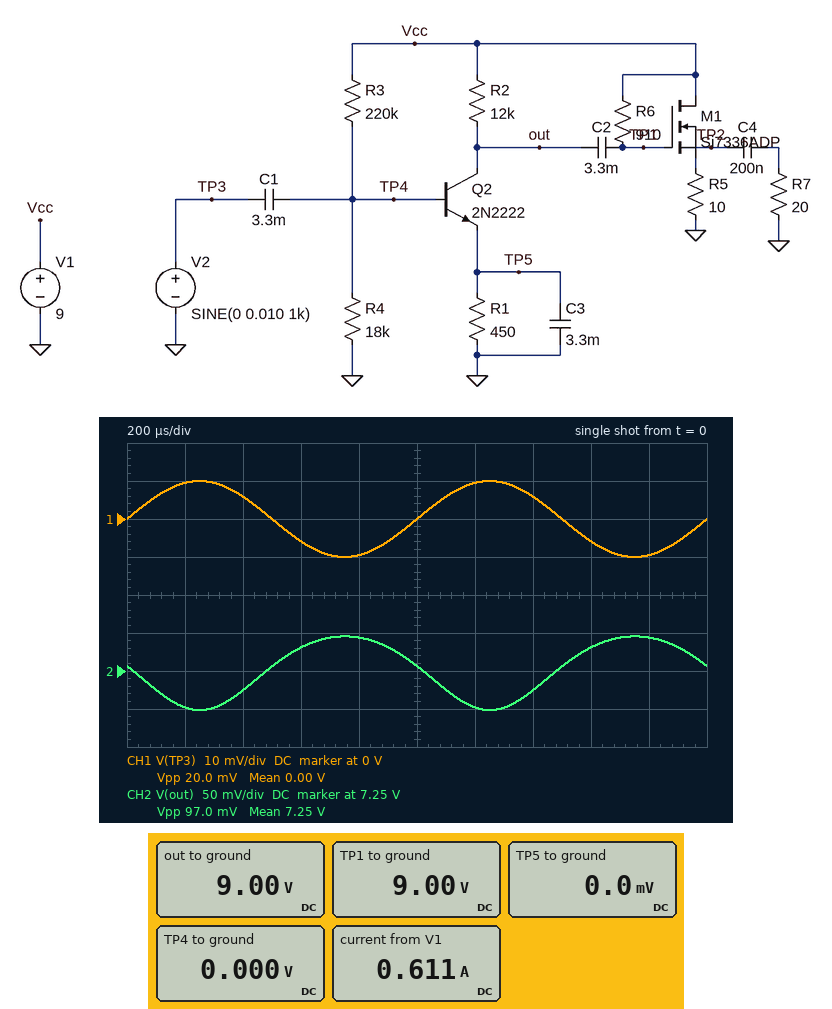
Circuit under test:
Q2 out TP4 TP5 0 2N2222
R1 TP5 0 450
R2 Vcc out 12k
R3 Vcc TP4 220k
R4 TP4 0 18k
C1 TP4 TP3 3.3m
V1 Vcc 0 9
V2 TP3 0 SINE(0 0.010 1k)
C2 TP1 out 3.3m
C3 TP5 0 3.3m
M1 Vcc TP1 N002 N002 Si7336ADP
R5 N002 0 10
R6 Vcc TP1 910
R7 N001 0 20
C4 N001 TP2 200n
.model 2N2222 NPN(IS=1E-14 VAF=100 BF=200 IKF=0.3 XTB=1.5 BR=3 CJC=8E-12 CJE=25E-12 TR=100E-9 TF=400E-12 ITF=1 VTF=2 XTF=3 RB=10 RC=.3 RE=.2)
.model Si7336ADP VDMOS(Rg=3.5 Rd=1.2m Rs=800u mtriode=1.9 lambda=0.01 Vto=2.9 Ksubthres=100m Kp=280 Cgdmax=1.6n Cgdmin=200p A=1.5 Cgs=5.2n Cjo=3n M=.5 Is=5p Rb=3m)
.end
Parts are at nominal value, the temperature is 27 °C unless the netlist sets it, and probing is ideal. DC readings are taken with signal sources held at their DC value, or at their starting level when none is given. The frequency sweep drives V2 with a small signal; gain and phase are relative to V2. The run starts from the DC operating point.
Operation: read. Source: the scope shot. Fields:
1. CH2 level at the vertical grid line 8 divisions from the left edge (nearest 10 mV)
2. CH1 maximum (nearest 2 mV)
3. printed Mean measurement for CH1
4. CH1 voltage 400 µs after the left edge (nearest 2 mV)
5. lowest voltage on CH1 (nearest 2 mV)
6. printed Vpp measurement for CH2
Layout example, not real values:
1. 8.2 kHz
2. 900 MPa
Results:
1. 7.28 V
2. 10 mV
3. 0.00 V
4. 6 mV
5. -10 mV
6. 97.0 mV
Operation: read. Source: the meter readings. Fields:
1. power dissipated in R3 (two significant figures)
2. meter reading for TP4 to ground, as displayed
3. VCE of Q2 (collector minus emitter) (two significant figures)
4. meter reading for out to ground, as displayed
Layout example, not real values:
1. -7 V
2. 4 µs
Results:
1. 370 µW
2. 0.000 V
3. 9.0 V
4. 9.00 V
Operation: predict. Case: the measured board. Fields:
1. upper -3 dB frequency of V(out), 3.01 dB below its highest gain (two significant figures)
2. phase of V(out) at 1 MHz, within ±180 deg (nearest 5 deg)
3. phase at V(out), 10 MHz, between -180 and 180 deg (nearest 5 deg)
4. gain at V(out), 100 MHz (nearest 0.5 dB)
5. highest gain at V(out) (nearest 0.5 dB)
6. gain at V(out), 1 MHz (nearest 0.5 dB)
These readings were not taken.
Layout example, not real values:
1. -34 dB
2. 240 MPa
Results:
1. 170 kHz
2. 100 deg
3. 100 deg
4. -34.0 dB
5. 13.5 dB
6. -2.0 dB
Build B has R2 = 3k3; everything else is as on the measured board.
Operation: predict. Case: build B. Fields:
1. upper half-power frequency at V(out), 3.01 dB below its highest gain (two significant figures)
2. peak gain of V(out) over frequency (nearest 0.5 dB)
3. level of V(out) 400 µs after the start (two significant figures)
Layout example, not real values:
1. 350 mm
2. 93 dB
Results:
1. 200 kHz
2. 12.0 dB
3. 8.5 V
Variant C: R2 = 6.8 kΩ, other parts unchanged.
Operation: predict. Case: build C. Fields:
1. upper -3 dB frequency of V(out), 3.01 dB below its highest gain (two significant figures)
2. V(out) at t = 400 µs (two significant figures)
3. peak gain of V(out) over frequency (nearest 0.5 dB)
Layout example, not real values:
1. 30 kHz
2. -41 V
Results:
1. 180 kHz
2. 8.0 V
3. 13.0 dB
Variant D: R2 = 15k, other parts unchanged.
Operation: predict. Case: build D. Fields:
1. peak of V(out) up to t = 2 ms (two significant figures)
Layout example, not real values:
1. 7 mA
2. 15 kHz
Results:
1. 6.9 V
